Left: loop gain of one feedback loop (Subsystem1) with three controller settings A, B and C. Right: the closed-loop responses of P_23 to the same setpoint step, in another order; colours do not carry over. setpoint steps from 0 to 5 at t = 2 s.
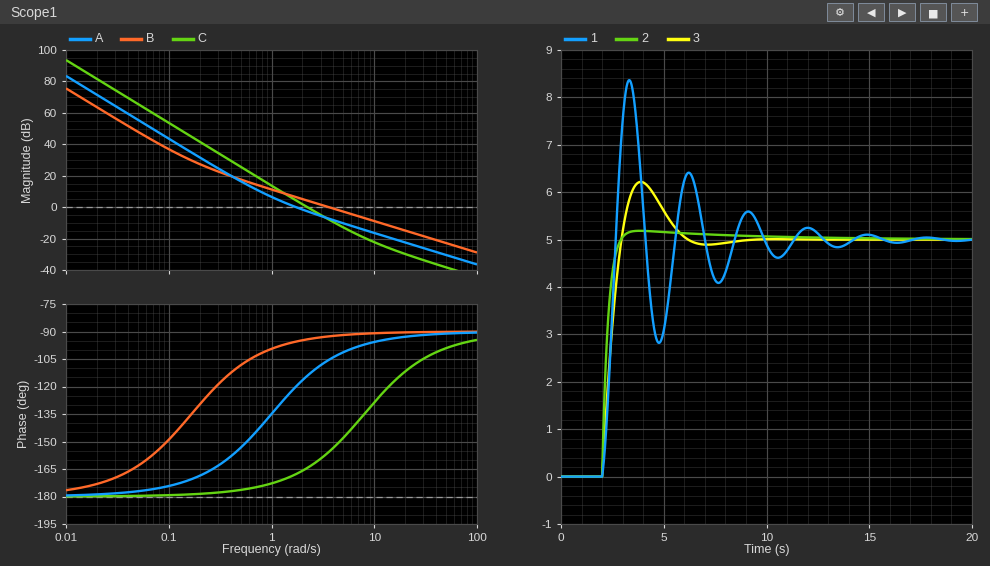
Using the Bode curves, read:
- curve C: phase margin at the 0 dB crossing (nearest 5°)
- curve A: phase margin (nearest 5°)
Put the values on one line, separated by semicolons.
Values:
15°; 60°
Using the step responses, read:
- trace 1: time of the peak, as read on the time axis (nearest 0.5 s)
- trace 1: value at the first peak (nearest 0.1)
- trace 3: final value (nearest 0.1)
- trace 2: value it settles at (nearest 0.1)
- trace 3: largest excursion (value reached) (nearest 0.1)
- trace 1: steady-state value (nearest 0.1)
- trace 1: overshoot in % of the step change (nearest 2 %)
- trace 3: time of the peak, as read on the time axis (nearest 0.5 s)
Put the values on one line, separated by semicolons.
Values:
3.5 s; 8.4; 5.0; 5.0; 6.2; 5.0; 68 %; 4.0 s
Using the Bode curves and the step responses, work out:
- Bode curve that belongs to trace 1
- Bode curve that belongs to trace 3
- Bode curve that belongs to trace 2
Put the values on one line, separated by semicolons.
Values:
C; A; B
